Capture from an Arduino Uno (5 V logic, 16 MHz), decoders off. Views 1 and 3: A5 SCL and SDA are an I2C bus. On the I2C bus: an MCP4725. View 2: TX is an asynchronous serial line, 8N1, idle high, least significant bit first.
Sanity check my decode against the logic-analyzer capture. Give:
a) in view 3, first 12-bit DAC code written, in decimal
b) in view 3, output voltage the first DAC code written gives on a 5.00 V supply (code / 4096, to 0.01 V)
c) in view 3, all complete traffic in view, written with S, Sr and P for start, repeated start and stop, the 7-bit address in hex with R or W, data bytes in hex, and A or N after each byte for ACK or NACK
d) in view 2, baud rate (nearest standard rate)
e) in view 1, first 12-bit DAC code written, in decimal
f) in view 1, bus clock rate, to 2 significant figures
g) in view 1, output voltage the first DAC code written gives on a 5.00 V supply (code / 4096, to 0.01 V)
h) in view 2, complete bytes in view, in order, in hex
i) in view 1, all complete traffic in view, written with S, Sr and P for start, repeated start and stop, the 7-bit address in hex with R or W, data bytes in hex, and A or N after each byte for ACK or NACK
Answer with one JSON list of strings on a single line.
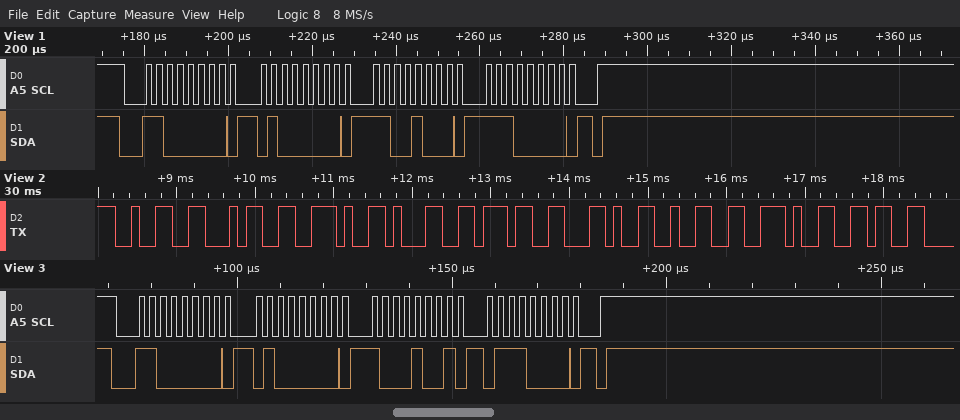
["2199", "2.68 V", "S 60W A 40 A 89 A 70 A P", "9600 baud", "3214", "400 kHz", "3.92 V", "32 34 2E 31 37 2C 32 2E 36", "S 60W A 40 A C8 A E0 A P"]
